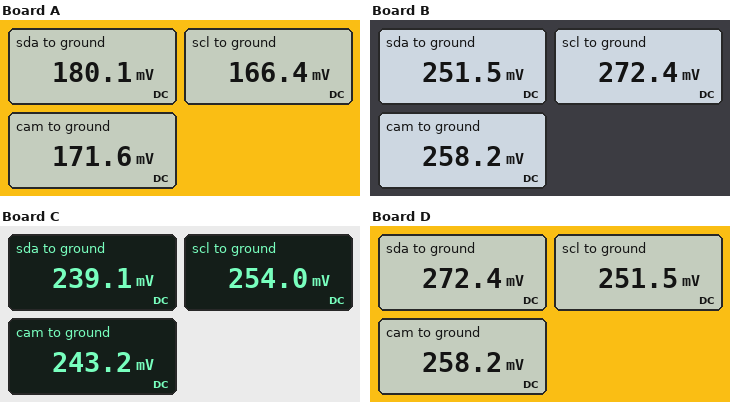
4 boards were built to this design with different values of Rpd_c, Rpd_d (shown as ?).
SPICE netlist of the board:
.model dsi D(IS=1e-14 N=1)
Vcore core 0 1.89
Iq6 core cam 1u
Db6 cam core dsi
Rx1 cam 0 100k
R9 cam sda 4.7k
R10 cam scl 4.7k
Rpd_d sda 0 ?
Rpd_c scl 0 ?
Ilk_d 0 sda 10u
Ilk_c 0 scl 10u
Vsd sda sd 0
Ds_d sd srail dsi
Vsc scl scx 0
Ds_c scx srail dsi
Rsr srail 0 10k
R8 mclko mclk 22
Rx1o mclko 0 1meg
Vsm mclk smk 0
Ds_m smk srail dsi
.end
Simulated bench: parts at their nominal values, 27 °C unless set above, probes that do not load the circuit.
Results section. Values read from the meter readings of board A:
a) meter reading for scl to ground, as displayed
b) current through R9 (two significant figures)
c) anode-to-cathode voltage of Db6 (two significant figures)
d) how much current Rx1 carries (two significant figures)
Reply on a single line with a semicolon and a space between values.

166.4 mV; 1.8 µA; -1.7 V; 1.7 µA
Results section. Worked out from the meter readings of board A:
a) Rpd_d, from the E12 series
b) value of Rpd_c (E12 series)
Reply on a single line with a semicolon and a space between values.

22 kΩ; 15 kΩ
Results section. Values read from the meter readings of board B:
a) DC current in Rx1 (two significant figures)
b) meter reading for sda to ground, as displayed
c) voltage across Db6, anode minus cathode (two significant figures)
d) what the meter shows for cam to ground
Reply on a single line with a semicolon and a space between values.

2.6 µA; 251.5 mV; -1.6 V; 258.2 mV
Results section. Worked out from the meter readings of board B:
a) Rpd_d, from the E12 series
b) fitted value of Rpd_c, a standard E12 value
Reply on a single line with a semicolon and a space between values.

22 kΩ; 39 kΩ
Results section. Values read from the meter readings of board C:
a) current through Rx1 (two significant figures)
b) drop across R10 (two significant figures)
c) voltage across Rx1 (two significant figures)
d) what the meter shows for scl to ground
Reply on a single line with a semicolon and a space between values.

2.4 µA; 11 mV; 240 mV; 254.0 mV
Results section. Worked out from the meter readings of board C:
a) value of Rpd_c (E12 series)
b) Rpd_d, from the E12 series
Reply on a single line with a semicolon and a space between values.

33 kΩ; 22 kΩ
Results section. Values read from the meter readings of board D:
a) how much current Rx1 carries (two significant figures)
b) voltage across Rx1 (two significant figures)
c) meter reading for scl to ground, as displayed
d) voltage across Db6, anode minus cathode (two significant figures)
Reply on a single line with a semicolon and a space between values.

2.6 µA; 260 mV; 251.5 mV; -1.6 V
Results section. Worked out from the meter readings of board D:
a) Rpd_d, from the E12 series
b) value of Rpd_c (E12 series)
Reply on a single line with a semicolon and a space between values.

39 kΩ; 22 kΩ
